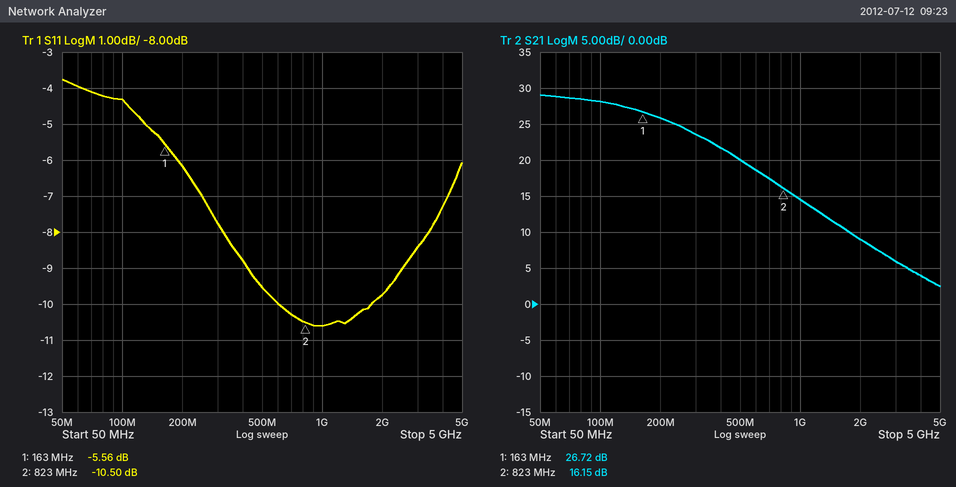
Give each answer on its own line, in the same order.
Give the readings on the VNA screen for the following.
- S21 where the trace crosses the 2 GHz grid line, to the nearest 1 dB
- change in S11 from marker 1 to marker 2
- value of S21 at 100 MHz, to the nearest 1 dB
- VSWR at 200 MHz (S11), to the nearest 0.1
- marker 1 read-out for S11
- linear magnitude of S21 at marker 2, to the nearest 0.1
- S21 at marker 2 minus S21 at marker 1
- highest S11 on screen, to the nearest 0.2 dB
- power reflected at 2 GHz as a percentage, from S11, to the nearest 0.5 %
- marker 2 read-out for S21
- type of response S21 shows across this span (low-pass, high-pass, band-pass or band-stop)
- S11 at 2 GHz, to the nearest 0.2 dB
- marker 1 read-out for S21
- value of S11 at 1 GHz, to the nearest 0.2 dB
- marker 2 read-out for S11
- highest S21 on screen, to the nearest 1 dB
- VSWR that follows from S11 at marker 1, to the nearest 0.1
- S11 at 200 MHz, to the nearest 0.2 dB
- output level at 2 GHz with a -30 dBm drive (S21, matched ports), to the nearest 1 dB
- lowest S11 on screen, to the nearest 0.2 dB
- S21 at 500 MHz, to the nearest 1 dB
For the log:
9 dB
-4.94 dB
28 dB
2.9
-5.56 dB
6.4
-10.57 dB
-3.8 dB
10.5 %
16.15 dB
low-pass
-9.8 dB
26.72 dB
-10.6 dB
-10.50 dB
29 dB
3.2
-6.2 dB
-21 dBm
-10.6 dB
20 dB
